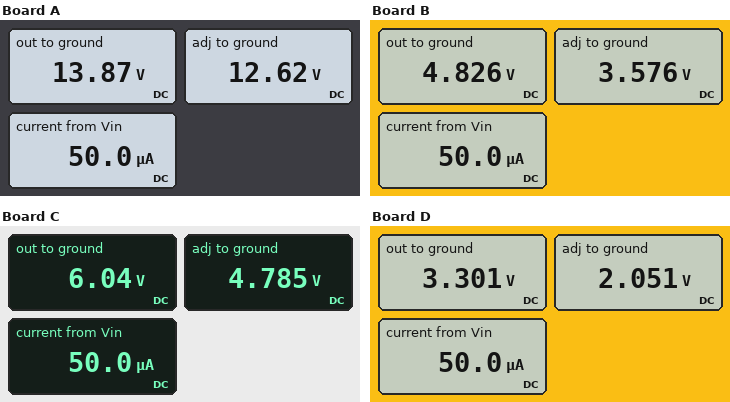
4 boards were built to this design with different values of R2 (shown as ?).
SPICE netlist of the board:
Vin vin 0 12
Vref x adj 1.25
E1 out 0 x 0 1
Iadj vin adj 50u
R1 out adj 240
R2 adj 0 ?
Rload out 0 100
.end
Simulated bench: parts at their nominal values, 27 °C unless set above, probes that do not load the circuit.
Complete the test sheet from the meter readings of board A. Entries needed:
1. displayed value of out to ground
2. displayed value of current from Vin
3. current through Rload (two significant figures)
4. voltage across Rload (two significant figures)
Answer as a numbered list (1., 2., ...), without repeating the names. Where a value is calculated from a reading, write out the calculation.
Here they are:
1. 13.87 V
2. 50.0 µA
3. (13.87 V) / 100 Ω = 140 mA
4. 13.87 V = 14 V
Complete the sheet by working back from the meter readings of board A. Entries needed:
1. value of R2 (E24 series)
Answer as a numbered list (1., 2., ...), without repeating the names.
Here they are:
1. 2.4 kΩ
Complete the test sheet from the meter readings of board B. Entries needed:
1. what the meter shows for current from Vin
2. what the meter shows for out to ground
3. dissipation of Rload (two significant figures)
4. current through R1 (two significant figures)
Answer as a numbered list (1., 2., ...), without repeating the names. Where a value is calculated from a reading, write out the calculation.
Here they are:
1. 50.0 µA
2. 4.826 V
3. (4.826 V)^2 / 100 Ω = 230 mW
4. (4.826 V - 3.576 V) / 240 Ω = 5.2 mA
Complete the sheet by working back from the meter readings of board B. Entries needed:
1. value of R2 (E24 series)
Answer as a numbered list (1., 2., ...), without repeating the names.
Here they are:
1. 680 Ω
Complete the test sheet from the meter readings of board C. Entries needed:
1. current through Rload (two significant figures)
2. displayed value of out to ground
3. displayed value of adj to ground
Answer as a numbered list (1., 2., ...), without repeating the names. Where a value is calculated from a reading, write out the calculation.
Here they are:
1. (6.04 V) / 100 Ω = 60 mA
2. 6.04 V
3. 4.785 V
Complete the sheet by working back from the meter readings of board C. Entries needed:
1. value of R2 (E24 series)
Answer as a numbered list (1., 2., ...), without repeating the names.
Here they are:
1. 910 Ω
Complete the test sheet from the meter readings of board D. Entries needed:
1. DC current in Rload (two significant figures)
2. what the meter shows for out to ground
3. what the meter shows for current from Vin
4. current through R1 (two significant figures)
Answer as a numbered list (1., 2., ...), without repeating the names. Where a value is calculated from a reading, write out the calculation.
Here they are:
1. (3.301 V) / 100 Ω = 33 mA
2. 3.301 V
3. 50.0 µA
4. (3.301 V - 2.051 V) / 240 Ω = 5.2 mA
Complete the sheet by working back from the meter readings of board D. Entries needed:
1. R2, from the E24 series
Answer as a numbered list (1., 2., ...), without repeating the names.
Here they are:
1. 390 Ω
